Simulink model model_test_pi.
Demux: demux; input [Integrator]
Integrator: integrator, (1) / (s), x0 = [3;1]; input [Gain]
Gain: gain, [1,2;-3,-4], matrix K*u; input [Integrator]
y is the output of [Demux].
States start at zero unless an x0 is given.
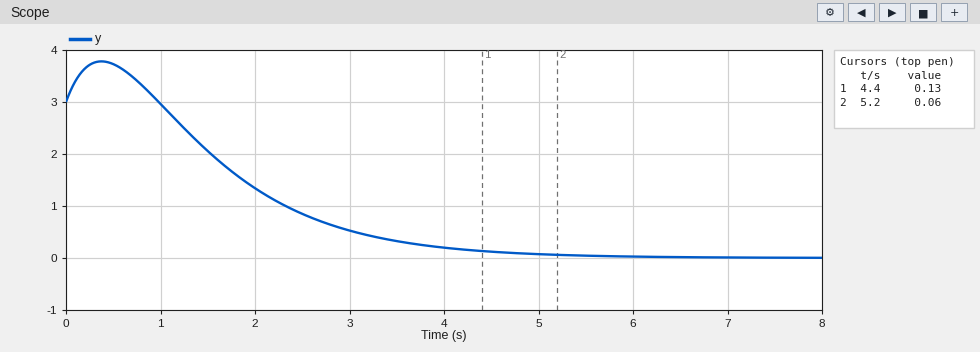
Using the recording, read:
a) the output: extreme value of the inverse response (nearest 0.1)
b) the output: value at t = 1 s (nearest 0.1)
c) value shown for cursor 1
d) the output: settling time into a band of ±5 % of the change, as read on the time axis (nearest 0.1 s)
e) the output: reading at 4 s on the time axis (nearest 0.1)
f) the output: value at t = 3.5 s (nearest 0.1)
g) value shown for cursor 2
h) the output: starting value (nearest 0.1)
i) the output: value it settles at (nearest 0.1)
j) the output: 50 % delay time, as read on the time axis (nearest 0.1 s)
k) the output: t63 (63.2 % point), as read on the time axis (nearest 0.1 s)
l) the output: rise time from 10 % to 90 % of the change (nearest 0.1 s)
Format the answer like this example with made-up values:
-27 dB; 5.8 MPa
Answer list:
3.8; 3.0; 0.13; 4.3 s; 0.2; 0.3; 0.06; 3.0; 0.0; 1.9 s; 2.2 s; 2.4 s
